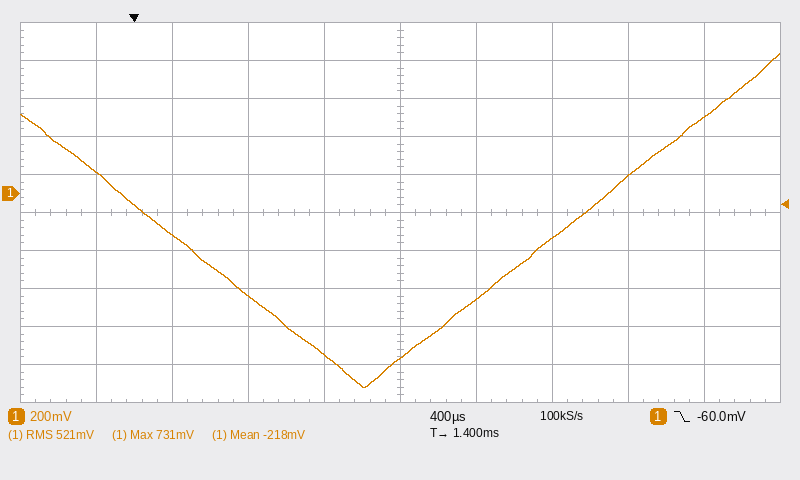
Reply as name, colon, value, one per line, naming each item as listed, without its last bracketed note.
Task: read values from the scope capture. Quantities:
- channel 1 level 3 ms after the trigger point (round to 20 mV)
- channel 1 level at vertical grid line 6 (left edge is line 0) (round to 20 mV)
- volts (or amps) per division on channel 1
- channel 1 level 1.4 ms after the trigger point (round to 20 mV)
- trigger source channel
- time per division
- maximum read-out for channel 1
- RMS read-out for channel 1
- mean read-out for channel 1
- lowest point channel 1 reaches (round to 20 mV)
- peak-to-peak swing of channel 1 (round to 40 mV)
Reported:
channel 1 level 3 ms after the trigger point: 400 mV
channel 1 level at vertical grid line 6 (left edge is line 0): -560 mV
volts (or amps) per division on channel 1: 200 mV
channel 1 level 1.4 ms after the trigger point: -860 mV
trigger source channel: channel 1
time per division: 400 µs
maximum read-out for channel 1: 731 mV
RMS read-out for channel 1: 521 mV
mean read-out for channel 1: -218 mV
lowest point channel 1 reaches: -1.02 V
peak-to-peak swing of channel 1: 1.76 V
